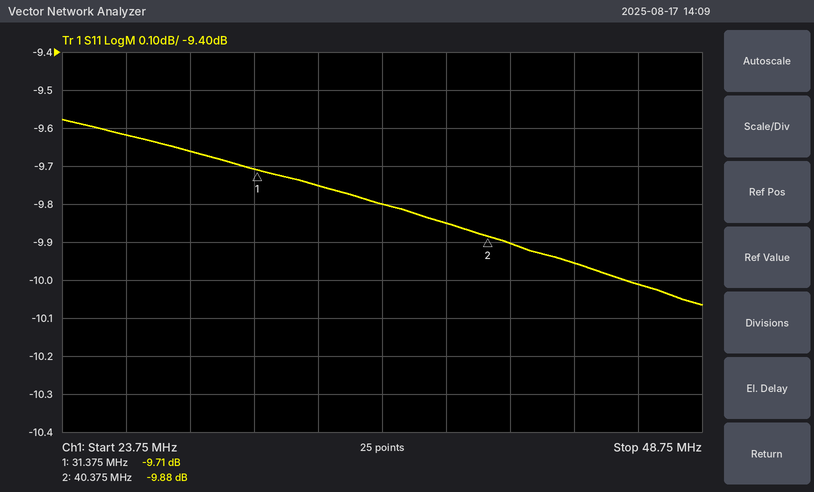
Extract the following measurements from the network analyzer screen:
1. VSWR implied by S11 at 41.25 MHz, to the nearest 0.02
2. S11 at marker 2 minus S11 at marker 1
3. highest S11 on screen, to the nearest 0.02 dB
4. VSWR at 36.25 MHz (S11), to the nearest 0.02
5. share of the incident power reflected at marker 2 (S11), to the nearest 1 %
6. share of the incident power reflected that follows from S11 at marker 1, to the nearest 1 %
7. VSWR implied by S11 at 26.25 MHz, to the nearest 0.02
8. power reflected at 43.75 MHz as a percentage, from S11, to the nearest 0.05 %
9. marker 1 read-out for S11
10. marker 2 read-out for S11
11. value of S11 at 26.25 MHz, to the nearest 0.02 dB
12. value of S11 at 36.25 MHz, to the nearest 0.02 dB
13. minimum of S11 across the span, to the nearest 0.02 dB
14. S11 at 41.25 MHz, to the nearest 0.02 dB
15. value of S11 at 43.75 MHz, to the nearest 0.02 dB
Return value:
1.94
-0.17 dB
-9.58 dB
1.96
10 %
11 %
1.98
10.10 %
-9.71 dB
-9.88 dB
-9.62 dB
-9.80 dB
-10.06 dB
-9.90 dB
-9.96 dB
